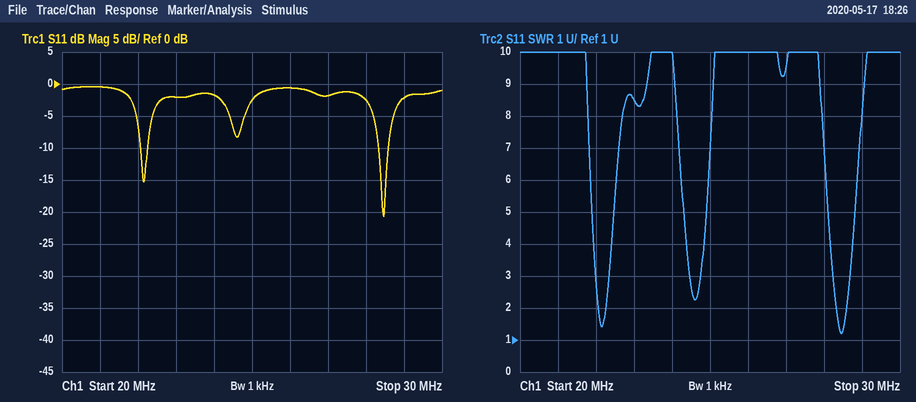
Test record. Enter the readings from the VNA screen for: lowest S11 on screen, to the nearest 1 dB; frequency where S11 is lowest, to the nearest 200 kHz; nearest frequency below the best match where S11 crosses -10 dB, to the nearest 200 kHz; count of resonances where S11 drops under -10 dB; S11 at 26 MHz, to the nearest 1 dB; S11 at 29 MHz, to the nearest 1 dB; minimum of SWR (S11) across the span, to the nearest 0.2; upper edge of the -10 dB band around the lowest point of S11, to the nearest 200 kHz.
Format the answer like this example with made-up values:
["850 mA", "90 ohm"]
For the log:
["-21 dB", "28.4 MHz", "28.4 MHz", "2", "-1 dB", "-2 dB", "1.2", "28.6 MHz"]
